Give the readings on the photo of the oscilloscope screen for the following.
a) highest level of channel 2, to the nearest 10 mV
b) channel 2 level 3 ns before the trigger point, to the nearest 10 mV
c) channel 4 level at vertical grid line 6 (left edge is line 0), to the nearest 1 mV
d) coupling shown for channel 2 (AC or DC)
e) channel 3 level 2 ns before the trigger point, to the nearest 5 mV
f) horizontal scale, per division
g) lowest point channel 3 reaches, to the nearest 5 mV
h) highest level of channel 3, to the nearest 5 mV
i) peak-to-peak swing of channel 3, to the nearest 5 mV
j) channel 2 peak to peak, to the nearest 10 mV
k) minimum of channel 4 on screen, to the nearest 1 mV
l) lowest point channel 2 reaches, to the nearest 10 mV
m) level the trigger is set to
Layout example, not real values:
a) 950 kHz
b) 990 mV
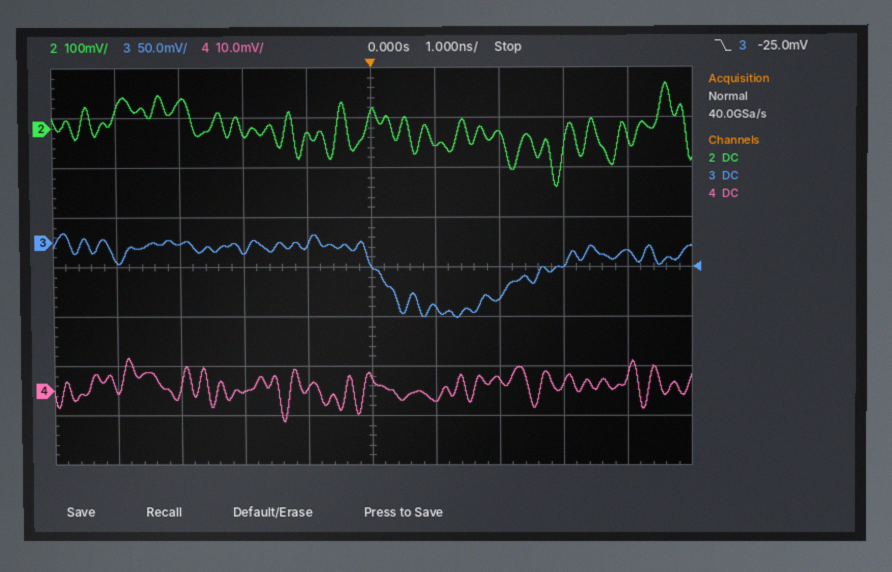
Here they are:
a) 90 mV
b) 50 mV
c) -2 mV
d) DC
e) -10 mV
f) 1 ns
g) -75 mV
h) 10 mV
i) 85 mV
j) 210 mV
k) -6 mV
l) -120 mV
m) -25.0 mV
